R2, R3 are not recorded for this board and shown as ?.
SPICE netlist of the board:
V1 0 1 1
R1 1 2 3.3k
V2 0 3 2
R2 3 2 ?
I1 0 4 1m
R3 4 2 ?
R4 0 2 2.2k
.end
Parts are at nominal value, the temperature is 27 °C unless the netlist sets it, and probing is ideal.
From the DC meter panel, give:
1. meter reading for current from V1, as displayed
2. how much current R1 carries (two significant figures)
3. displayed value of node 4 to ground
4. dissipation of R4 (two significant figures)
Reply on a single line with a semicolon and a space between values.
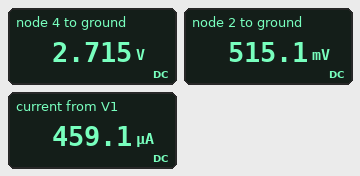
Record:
459.1 µA; 460 µA; 2.715 V; 120 µW
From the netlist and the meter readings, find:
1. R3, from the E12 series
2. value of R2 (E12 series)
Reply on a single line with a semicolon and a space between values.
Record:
2.2 kΩ; 8.2 kΩ
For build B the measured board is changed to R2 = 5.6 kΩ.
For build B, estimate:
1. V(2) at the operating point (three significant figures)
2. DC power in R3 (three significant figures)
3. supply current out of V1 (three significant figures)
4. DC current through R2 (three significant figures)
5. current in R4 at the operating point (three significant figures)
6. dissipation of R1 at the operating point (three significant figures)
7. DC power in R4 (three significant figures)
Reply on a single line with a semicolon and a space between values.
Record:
363 mV; 2.20 mW; 413 µA; 422 µA; 165 µA; 563 µW; 59.9 µW
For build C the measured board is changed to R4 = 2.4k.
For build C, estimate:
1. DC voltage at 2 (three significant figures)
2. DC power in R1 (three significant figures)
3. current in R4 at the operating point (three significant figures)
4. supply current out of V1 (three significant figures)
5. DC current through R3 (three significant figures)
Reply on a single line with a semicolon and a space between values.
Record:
538 mV; 717 µW; 224 µA; 466 µA; 1.00 mA
